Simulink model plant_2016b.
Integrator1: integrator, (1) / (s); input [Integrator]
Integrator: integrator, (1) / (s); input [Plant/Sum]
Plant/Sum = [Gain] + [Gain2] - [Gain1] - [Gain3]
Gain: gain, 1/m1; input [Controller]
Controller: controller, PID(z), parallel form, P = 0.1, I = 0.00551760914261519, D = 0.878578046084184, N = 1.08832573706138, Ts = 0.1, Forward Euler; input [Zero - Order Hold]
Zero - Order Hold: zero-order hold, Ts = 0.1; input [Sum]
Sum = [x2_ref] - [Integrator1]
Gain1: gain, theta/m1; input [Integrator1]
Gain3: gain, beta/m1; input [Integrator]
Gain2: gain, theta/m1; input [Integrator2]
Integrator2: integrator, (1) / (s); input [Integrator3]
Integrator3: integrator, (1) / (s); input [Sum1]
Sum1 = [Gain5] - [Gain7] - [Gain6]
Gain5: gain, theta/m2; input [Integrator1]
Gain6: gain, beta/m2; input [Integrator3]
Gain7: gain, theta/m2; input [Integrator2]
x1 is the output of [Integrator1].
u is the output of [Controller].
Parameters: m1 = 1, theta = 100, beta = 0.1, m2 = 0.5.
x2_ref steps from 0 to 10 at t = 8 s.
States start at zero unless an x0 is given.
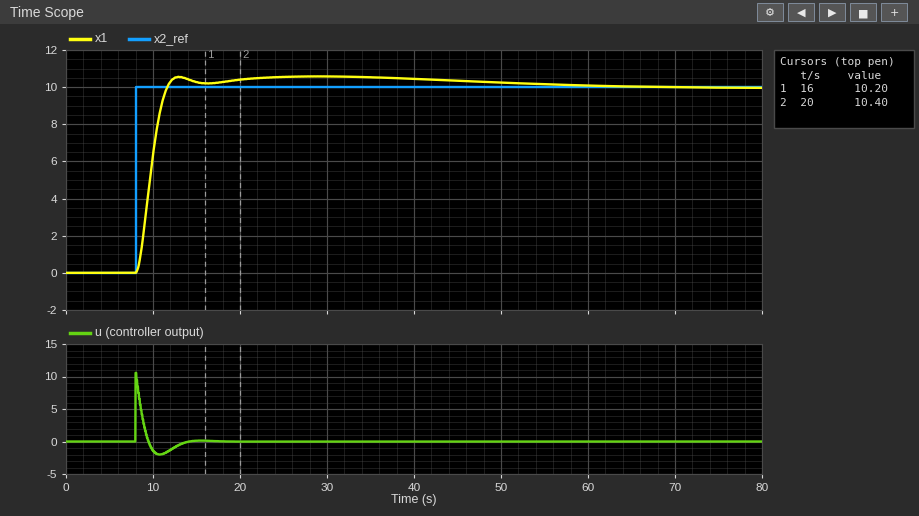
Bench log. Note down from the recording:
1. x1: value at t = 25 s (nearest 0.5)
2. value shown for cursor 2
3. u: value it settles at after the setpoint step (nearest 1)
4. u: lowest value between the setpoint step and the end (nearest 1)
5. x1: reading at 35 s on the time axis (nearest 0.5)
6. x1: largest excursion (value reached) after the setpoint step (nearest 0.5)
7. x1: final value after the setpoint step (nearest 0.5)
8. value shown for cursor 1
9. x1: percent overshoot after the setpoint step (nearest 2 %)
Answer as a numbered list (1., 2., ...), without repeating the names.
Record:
1. 10.5
2. 10.40
3. 0
4. -2
5. 10.5
6. 10.5
7. 10.0
8. 10.20
9. 6 %
